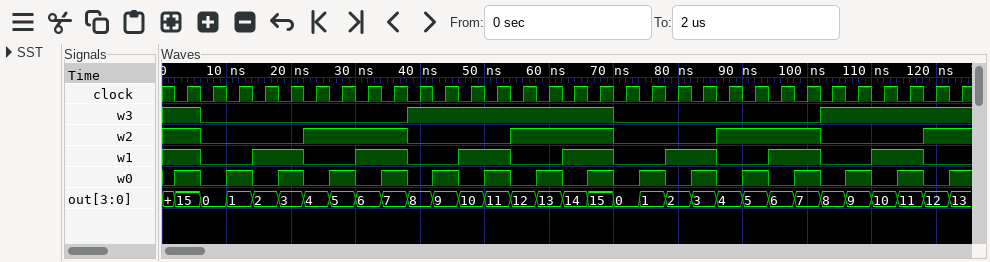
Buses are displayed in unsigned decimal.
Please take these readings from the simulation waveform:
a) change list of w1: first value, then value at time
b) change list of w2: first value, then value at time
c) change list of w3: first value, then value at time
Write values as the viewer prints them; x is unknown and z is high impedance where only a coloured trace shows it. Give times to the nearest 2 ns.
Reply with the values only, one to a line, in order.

1, 0 at 6 ns, 1 at 14 ns, 0 at 22 ns, 1 at 30 ns, 0 at 38 ns, 1 at 46 ns, 0 at 54 ns, 1 at 62 ns, 0 at 70 ns, 1 at 78 ns, 0 at 86 ns, 1 at 94 ns, 0 at 102 ns, 1 at 110 ns, 0 at 118 ns
1, 0 at 6 ns, 1 at 22 ns, 0 at 38 ns, 1 at 54 ns, 0 at 70 ns, 1 at 86 ns, 0 at 102 ns, 1 at 118 ns
1, 0 at 6 ns, 1 at 38 ns, 0 at 70 ns, 1 at 102 ns
